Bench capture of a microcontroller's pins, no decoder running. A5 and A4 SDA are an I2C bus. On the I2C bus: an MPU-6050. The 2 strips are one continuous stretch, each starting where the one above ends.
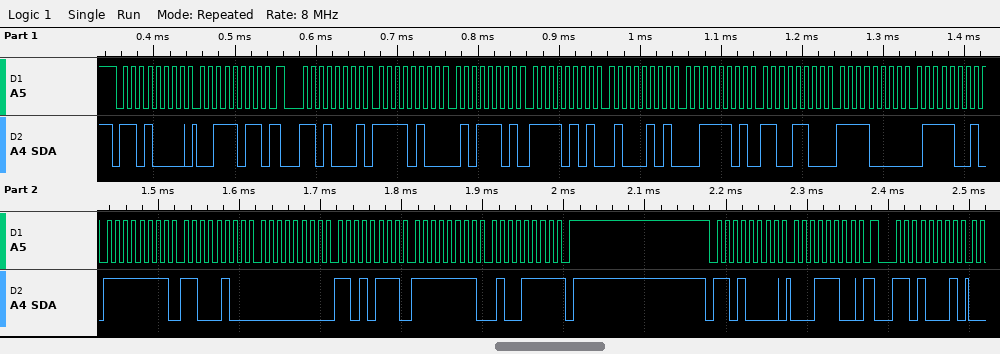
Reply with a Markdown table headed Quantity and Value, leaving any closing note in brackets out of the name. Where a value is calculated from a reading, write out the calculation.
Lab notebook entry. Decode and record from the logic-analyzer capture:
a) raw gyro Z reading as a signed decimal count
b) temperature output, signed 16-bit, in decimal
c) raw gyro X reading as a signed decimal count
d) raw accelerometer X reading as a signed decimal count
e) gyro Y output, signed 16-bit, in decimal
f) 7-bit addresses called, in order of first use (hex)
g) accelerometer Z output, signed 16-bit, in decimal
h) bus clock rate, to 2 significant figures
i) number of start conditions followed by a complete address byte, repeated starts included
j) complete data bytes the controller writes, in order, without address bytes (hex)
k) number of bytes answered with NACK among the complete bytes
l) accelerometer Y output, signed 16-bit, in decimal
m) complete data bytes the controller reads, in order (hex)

| Quantity | Value |
|---|---|
| raw gyro Z reading as a signed decimal count | 0xFF4F = -177 |
| temperature output, signed 16-bit, in decimal | 0xF079 = -3975 |
| raw gyro X reading as a signed decimal count | 0xFFC4 = -60 |
| raw accelerometer X reading as a signed decimal count | 0xF45D = -2979 |
| gyro Y output, signed 16-bit, in decimal | 0x00D7 = 215 |
| 7-bit addresses called, in order of first use | 0x68 |
| accelerometer Z output, signed 16-bit, in decimal | 0x3DCC = 15820 |
| bus clock rate, to 2 significant figures | 100 kHz |
| number of start conditions followed by a complete address byte, repeated starts included | 4 |
| complete data bytes the controller writes, in order, without address bytes | 3B 1C |
| number of bytes answered with NACK among the complete bytes | 1 |
| accelerometer Y output, signed 16-bit, in decimal | 0xF545 = -2747 |
| complete data bytes the controller reads, in order | F4 5D F5 45 3D CC F0 79 FF C4 00 D7 FF 4F |
